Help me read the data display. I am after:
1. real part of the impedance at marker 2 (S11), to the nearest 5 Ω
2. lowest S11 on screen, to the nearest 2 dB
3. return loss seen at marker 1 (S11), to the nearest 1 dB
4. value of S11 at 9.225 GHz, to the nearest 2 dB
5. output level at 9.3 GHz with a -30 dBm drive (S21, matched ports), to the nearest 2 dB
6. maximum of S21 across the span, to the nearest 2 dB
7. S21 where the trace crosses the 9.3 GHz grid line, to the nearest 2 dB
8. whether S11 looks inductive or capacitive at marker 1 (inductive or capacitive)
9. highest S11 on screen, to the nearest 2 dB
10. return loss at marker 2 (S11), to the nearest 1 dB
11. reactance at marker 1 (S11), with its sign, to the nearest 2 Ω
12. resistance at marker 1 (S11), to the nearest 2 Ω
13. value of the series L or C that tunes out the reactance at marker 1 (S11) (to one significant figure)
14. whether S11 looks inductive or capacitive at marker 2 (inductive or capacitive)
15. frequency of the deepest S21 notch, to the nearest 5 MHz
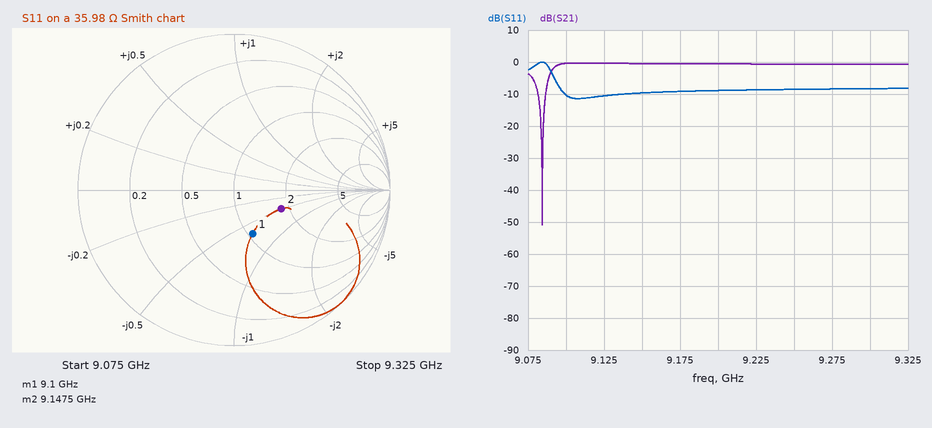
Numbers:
65 Ω
-12 dB
10 dB
-8 dB
-30 dBm
0 dB
0 dB
capacitive
0 dB
10 dB
-24 Ω
38 Ω
400 pH
capacitive
9.085 GHz
